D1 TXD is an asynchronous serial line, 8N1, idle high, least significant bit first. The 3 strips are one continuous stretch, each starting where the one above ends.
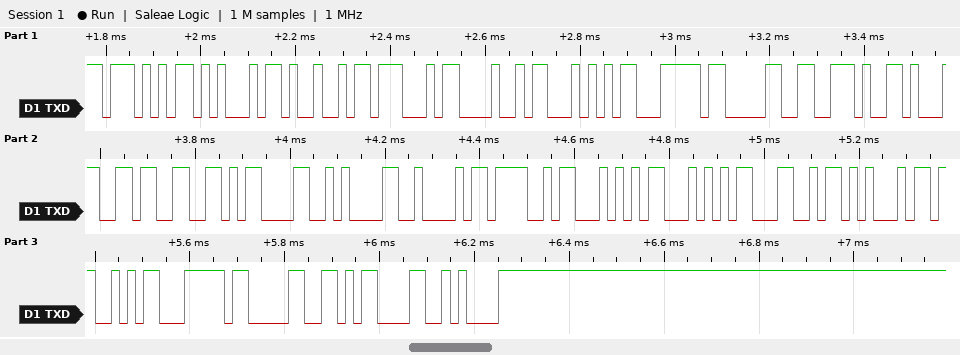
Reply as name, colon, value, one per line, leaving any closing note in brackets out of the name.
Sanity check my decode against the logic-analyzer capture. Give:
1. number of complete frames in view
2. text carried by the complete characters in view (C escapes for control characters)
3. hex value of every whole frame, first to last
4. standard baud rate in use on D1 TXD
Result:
number of complete frames in view: 24
text carried by the complete characters in view: "WEIGHT|0.13\r\nBOTTLES|0\r\n"
hex value of every whole frame, first to last: 57 45 49 47 48 54 7C 30 2E 31 33 0D 0A 42 4F 54 54 4C 45 53 7C 30 0D 0A
standard baud rate in use on D1 TXD: 57600 baud
